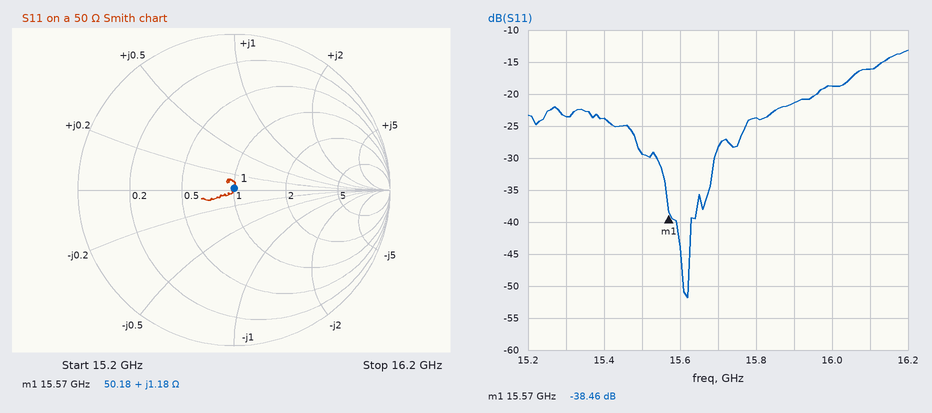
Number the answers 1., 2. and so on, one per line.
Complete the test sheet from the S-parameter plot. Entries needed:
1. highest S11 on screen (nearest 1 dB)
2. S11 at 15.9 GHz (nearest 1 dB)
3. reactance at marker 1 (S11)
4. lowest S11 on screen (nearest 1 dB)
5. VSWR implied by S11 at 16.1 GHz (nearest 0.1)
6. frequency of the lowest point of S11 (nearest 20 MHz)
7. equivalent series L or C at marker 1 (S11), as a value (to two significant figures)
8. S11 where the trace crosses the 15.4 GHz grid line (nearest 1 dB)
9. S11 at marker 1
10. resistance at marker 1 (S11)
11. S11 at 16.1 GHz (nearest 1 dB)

1. -13 dB
2. -21 dB
3. +1.18 Ω
4. -52 dB
5. 1.4
6. 15.62 GHz
7. 12 pH
8. -24 dB
9. -38.46 dB
10. 50.18 Ω
11. -16 dB
